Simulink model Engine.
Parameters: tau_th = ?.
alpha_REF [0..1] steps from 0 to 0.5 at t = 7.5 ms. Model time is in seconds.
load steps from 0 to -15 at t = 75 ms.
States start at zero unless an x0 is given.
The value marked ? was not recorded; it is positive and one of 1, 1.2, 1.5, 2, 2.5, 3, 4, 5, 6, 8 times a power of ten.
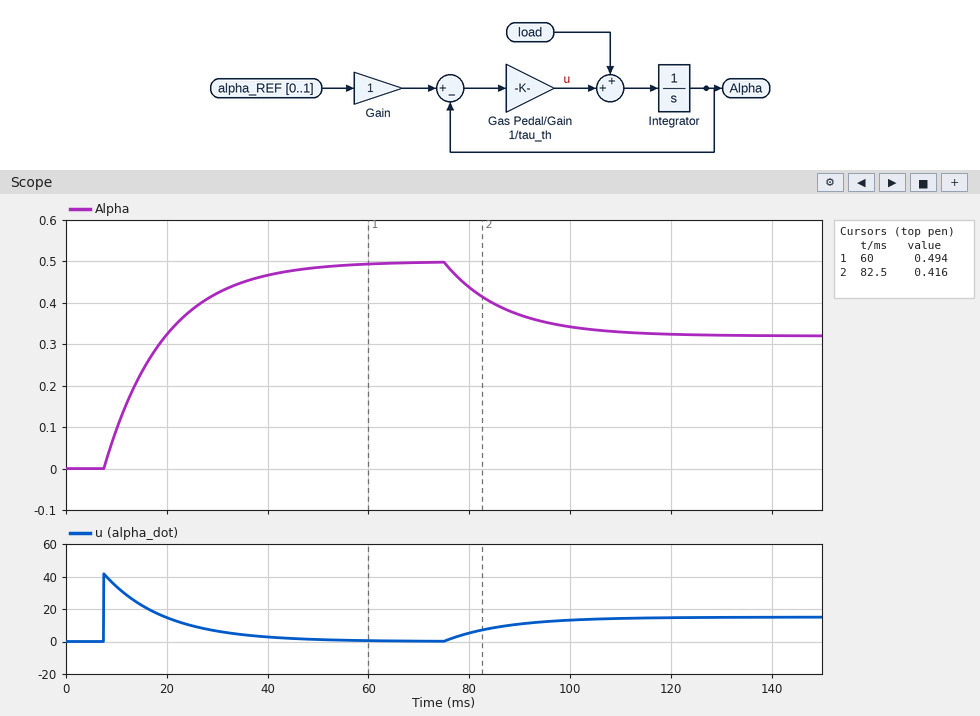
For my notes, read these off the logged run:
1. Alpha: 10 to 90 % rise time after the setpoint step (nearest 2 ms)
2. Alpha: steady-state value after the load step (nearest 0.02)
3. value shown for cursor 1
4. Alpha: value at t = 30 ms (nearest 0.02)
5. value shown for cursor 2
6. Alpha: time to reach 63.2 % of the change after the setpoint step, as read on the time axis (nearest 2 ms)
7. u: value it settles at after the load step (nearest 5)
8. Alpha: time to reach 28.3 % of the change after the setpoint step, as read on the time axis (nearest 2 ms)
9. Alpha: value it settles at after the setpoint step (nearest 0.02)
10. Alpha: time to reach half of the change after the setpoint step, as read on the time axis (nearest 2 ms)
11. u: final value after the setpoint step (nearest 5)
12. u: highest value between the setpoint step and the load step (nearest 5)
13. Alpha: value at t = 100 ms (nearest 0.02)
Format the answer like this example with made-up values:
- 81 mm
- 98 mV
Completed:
- 26 ms
- 0.32
- 0.494
- 0.42
- 0.416
- 20 ms
- 15
- 12 ms
- 0.50
- 16 ms
- 0
- 40
- 0.34
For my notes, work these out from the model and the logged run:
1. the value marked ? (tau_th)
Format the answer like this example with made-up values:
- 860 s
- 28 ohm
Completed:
- 0.012
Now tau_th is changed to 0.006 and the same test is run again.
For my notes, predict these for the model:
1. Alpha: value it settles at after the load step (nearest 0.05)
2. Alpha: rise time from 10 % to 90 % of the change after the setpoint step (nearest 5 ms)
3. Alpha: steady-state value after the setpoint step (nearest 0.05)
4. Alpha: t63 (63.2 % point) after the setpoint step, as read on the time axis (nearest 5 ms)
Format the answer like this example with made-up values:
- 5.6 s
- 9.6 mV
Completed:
- 0.40
- 15 ms
- 0.50
- 15 ms
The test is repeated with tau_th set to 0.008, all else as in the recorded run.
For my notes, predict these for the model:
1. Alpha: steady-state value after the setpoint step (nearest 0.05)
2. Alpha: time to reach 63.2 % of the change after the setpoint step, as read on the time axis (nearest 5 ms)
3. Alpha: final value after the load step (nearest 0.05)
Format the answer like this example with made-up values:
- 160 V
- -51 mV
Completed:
- 0.50
- 15 ms
- 0.40
